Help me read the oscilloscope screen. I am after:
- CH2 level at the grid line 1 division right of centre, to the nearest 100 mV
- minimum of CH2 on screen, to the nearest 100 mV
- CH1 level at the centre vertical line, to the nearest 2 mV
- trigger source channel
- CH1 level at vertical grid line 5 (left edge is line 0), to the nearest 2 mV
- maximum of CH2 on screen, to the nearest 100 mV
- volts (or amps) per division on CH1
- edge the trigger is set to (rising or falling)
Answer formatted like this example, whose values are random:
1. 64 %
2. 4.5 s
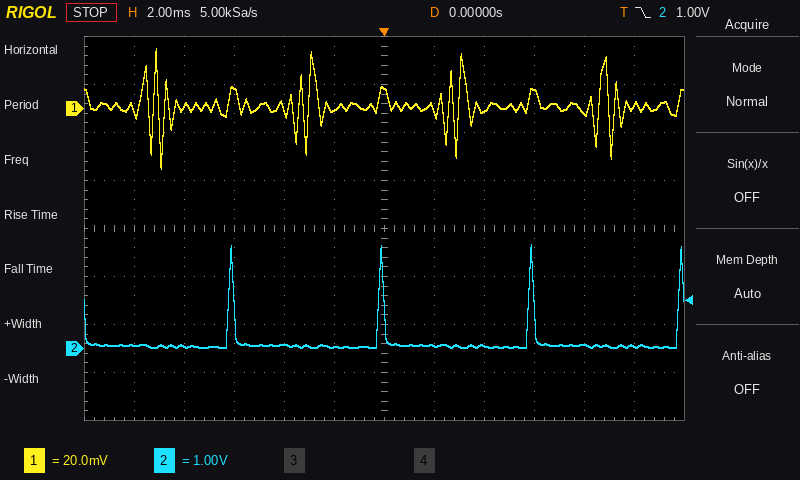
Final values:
1. 100 mV
2. 0.0 V
3. 8 mV
4. CH2
5. 0 mV
6. 2.2 V
7. 20 mV
8. falling
